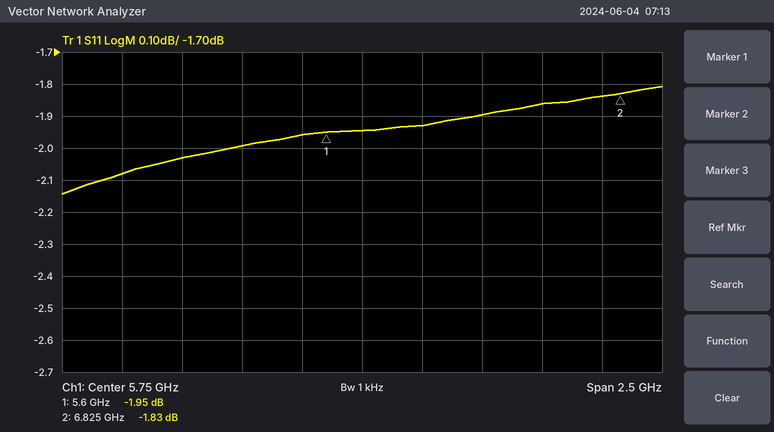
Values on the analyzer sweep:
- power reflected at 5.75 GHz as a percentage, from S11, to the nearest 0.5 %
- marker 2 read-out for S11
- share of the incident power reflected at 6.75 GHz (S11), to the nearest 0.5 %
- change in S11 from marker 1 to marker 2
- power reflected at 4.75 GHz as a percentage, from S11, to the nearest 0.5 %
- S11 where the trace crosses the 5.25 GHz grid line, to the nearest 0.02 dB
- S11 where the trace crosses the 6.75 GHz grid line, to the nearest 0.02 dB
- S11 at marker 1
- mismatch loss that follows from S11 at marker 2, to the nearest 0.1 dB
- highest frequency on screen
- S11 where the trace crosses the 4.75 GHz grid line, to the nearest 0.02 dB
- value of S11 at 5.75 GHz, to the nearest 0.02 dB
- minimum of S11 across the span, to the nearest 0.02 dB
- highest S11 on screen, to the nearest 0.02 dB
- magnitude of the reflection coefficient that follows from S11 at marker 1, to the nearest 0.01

64.0 %
-1.83 dB
65.5 %
0.12 dB
62.0 %
-2.00 dB
-1.84 dB
-1.95 dB
4.6 dB
7 GHz
-2.08 dB
-1.94 dB
-2.14 dB
-1.80 dB
0.80
